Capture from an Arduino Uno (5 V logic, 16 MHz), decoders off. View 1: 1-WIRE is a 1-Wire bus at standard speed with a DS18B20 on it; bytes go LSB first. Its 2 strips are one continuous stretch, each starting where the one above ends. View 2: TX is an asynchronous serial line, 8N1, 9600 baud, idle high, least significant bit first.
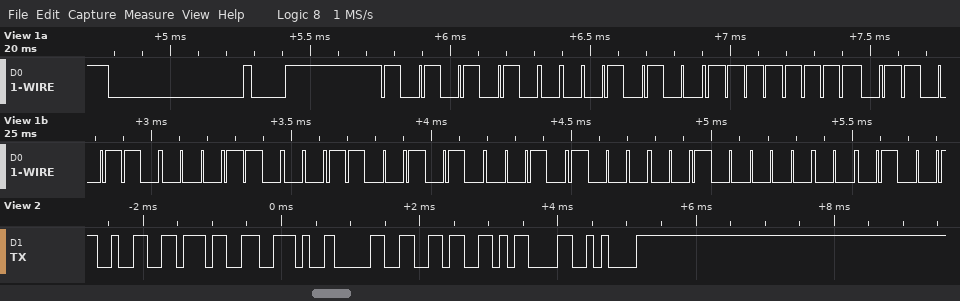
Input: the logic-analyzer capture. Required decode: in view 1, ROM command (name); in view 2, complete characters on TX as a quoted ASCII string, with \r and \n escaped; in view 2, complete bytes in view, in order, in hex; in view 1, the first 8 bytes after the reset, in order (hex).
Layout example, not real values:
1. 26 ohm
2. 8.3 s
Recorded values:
1. Match ROM
2. "27.06\r\n"
3. 32 37 2E 30 36 0D 0A
4. 55 28 FF 66 18 53 14 04
